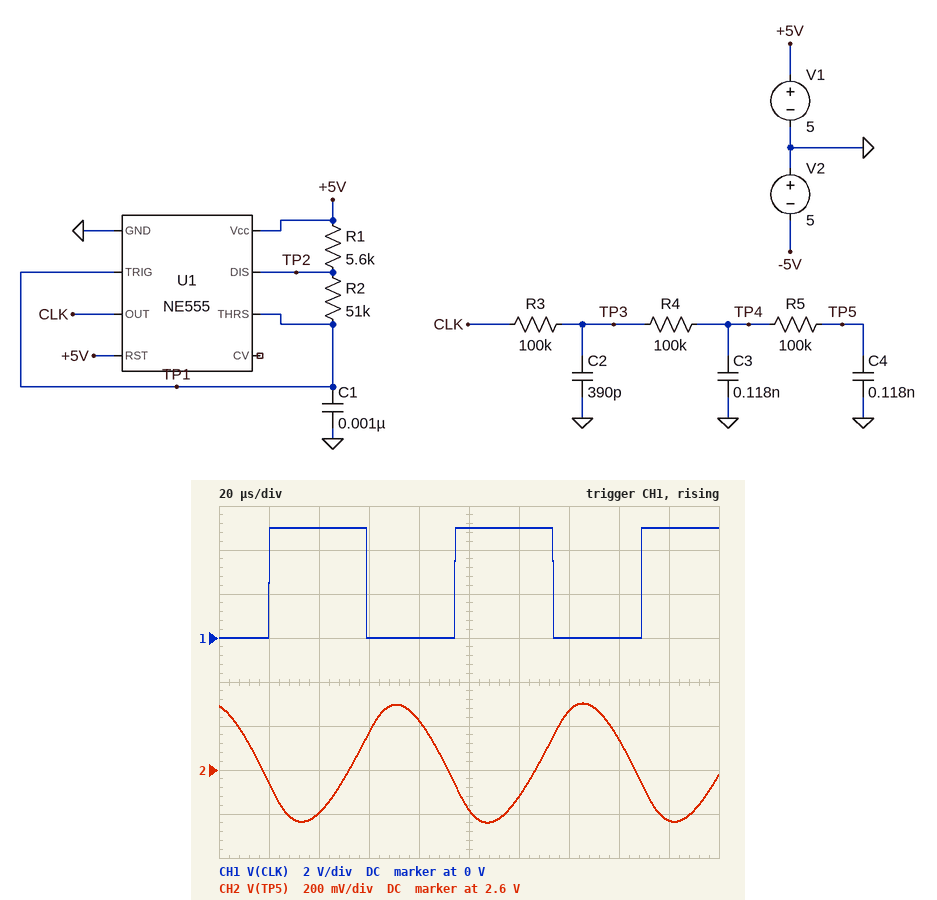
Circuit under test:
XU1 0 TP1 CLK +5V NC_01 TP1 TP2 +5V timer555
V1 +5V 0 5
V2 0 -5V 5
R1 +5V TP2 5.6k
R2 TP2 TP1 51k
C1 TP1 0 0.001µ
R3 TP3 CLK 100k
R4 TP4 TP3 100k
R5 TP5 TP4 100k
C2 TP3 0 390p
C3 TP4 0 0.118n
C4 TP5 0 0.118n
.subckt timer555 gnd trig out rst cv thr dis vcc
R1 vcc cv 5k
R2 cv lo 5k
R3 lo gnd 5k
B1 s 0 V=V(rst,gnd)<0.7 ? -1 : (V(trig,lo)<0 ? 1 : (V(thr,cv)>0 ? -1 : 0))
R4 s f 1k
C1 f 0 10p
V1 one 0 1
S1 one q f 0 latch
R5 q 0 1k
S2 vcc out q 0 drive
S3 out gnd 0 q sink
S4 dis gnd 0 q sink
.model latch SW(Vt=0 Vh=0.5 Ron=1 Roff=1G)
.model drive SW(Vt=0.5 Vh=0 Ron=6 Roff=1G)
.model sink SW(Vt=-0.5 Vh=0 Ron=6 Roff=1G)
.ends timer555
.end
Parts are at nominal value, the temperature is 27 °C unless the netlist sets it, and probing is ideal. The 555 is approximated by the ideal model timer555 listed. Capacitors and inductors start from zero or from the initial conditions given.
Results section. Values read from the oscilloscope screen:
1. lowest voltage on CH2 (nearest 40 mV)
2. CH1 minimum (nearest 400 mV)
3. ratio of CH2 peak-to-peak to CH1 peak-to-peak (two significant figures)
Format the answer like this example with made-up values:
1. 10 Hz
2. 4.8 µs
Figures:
1. 2.36 V
2. 0 V
3. 0.11
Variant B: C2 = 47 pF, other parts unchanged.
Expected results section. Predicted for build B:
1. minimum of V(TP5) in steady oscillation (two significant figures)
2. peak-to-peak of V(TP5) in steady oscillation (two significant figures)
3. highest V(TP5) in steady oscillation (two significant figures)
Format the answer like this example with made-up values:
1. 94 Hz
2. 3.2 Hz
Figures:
1. 2.0 V
2. 1.3 V
3. 3.3 V
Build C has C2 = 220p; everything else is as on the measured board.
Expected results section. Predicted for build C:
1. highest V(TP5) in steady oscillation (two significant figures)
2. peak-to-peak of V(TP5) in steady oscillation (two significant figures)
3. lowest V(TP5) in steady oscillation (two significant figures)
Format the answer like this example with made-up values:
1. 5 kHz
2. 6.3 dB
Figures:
1. 3.0 V
2. 800 mV
3. 2.2 V
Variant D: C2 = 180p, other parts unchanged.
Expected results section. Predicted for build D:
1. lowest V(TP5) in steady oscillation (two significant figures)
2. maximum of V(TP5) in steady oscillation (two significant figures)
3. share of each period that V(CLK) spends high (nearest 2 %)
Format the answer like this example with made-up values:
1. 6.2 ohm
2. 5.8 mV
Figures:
1. 2.2 V
2. 3.1 V
3. 52 %
